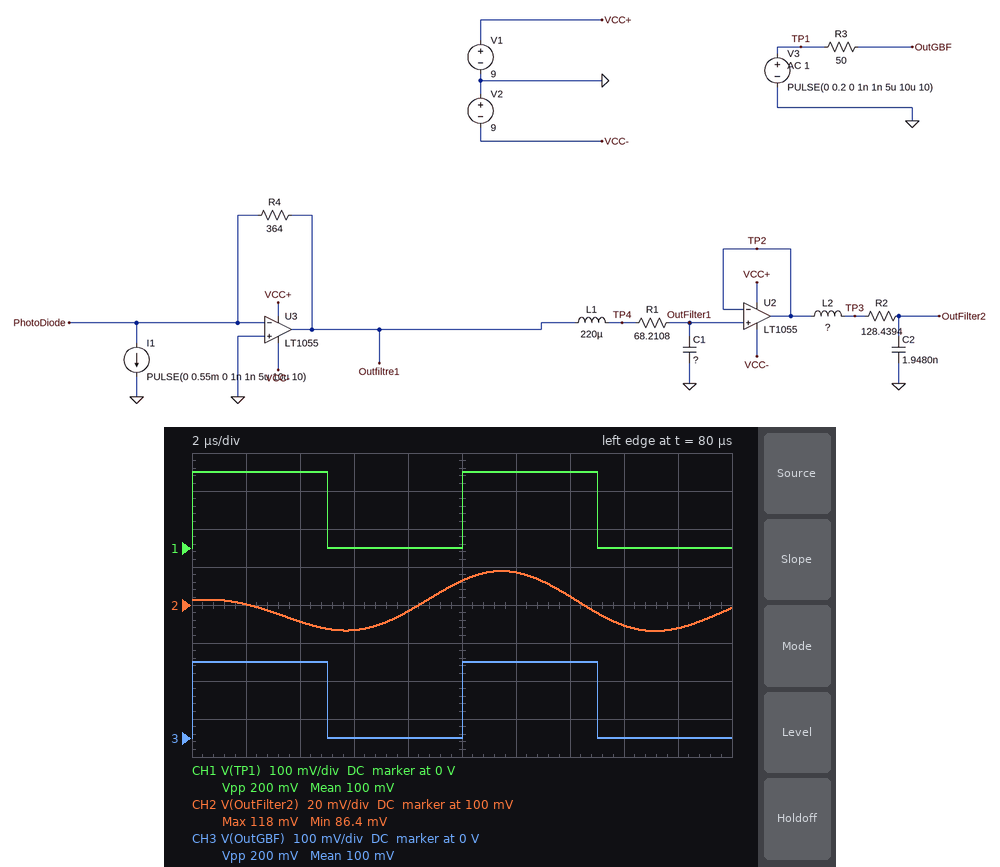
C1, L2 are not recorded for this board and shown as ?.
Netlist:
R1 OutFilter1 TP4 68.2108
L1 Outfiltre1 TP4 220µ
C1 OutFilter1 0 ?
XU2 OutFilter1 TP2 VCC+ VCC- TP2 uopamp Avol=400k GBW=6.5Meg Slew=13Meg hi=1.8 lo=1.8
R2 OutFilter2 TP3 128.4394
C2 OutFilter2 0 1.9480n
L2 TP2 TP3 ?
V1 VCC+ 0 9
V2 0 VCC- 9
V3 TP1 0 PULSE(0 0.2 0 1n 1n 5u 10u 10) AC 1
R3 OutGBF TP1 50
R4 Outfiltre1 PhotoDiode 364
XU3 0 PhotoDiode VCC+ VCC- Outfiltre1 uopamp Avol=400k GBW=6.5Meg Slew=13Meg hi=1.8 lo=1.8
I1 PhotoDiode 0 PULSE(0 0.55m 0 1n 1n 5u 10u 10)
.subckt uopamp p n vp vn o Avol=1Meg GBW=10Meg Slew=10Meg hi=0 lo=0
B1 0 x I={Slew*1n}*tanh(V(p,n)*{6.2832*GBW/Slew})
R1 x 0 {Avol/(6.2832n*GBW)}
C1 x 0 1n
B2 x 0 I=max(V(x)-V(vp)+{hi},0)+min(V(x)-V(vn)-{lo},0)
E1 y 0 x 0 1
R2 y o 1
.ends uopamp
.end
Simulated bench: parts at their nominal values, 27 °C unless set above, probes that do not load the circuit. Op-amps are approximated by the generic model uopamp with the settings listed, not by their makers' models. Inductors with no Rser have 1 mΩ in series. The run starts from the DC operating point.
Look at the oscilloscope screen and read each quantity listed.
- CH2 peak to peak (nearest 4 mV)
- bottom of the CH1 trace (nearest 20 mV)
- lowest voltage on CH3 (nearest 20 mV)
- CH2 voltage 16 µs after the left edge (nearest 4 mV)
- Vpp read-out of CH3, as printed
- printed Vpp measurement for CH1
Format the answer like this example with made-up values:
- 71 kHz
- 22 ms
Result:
- 32 mV
- 0 V
- 0 V
- 88 mV
- 200 mV
- 200 mV
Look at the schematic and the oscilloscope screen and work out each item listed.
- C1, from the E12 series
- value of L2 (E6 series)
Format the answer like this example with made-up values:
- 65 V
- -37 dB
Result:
- 100 nF
- 3.3 mH
